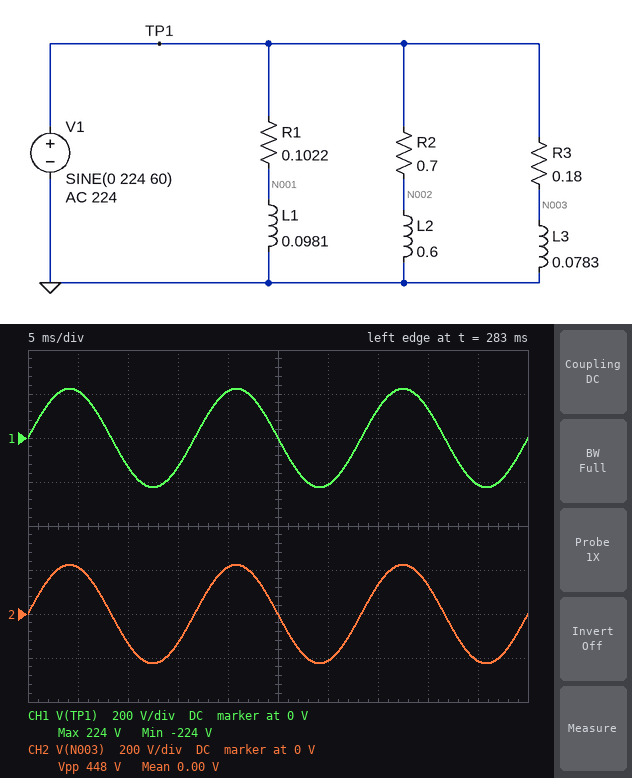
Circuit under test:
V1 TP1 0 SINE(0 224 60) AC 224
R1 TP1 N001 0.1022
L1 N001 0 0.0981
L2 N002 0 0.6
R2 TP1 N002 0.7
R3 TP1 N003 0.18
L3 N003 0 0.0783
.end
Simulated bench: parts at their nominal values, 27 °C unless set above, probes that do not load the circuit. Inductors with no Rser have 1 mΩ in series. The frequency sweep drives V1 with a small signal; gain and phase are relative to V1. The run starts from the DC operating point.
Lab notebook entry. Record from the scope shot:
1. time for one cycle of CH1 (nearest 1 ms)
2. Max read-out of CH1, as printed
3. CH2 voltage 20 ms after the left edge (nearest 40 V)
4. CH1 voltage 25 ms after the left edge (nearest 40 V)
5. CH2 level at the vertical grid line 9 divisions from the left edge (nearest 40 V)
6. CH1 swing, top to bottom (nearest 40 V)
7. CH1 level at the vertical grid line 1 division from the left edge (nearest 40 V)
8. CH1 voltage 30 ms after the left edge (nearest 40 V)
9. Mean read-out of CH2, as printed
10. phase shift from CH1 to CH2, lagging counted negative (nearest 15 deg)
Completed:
17 ms
224 V
200 V
0 V
-200 V
440 V
200 V
-200 V
0.00 V
0 deg
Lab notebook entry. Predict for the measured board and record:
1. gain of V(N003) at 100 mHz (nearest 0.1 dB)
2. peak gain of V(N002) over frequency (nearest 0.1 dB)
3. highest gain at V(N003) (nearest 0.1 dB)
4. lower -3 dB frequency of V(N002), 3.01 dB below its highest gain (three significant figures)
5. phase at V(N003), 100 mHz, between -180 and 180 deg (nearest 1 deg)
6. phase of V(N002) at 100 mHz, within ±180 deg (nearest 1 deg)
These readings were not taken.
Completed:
-11.6 dB
0 dB
0 dB
186 mHz
74 deg
62 deg
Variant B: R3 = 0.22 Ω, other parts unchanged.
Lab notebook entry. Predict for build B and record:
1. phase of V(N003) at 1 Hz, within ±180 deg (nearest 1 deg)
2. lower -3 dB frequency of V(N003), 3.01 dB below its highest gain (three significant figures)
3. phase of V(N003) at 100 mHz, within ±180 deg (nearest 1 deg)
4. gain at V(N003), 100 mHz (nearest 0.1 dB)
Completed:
24 deg
449 mHz
76 deg
-13.3 dB
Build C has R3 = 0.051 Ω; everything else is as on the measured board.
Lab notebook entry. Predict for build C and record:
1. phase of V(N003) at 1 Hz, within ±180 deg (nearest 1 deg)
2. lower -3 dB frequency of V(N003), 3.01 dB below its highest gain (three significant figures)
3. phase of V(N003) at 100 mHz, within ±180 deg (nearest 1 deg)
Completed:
6 deg
106 mHz
45 deg
